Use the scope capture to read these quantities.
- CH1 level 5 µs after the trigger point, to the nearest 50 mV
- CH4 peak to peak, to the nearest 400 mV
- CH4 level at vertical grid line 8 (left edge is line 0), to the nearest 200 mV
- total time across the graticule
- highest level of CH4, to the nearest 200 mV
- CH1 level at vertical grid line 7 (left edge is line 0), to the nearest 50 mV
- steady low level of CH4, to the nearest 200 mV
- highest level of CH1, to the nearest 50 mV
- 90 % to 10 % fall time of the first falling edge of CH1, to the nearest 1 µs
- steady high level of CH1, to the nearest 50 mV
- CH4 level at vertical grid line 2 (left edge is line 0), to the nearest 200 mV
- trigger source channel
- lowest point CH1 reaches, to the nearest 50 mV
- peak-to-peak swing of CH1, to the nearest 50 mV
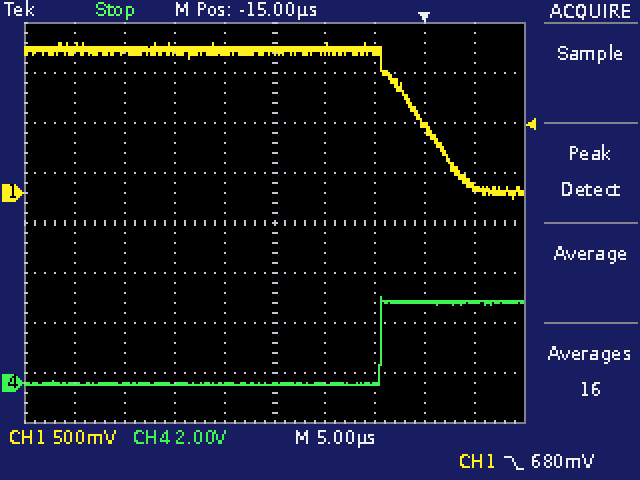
50 mV
3.6 V
3.2 V
50 µs
3.4 V
1.40 V
0.0 V
1.50 V
8 µs
1.40 V
0.0 V
CH1
-50 mV
1.55 V
